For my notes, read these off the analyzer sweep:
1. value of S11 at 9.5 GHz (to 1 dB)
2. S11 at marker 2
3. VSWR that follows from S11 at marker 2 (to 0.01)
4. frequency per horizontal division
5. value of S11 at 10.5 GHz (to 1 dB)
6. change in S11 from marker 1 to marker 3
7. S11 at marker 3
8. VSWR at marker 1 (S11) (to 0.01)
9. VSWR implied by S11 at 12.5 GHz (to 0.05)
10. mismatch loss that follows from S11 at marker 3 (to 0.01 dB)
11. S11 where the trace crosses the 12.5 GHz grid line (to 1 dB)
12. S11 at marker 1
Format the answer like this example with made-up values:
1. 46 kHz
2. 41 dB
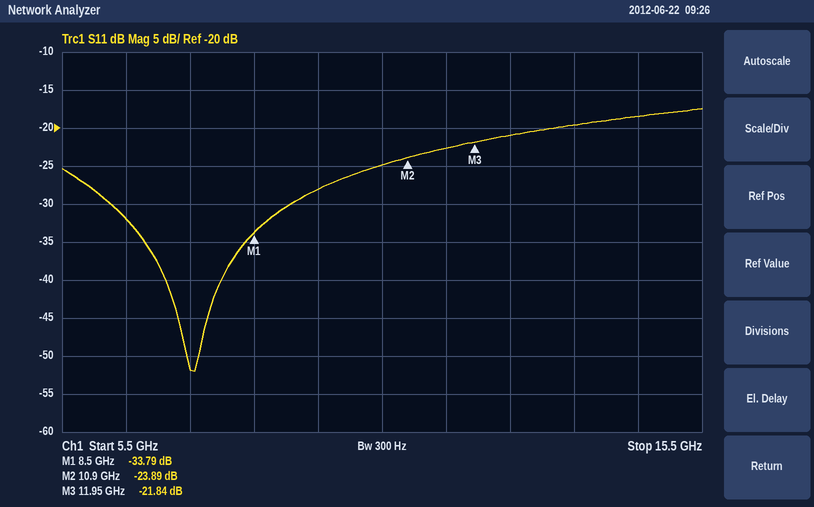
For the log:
1. -28 dB
2. -23.89 dB
3. 1.14
4. 1 GHz
5. -25 dB
6. 11.95 dB
7. -21.84 dB
8. 1.04
9. 1.20
10. 0.03 dB
11. -21 dB
12. -33.79 dB
